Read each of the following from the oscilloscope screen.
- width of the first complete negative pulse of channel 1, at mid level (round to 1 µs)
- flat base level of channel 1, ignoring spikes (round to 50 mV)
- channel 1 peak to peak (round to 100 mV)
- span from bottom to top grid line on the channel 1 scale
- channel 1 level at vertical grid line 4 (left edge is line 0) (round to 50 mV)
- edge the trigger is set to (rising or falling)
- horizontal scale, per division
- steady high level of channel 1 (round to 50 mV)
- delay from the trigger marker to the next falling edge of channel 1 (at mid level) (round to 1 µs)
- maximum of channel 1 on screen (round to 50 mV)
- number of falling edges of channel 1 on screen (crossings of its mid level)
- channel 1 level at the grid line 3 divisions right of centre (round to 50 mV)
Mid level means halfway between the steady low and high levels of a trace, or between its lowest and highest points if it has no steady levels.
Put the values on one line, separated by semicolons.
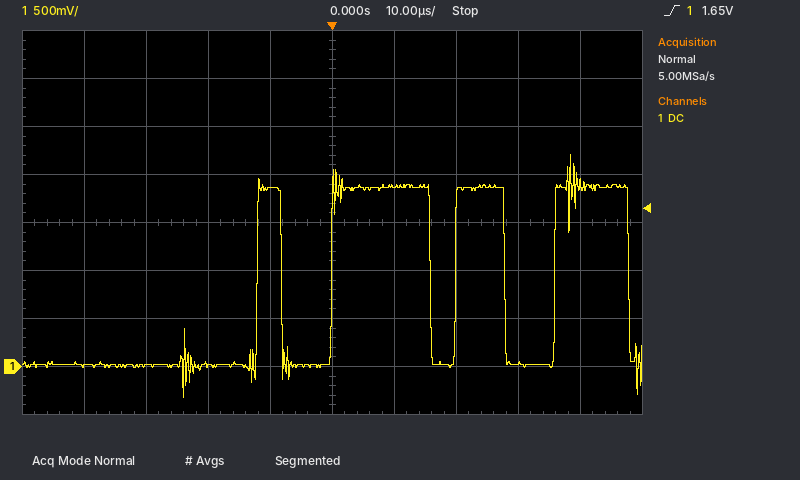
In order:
8 µs; 0 mV; 2.50 V; 4 V; 1.85 V; rising; 10 µs; 1.85 V; 16 µs; 2.20 V; 4; 50 mV
